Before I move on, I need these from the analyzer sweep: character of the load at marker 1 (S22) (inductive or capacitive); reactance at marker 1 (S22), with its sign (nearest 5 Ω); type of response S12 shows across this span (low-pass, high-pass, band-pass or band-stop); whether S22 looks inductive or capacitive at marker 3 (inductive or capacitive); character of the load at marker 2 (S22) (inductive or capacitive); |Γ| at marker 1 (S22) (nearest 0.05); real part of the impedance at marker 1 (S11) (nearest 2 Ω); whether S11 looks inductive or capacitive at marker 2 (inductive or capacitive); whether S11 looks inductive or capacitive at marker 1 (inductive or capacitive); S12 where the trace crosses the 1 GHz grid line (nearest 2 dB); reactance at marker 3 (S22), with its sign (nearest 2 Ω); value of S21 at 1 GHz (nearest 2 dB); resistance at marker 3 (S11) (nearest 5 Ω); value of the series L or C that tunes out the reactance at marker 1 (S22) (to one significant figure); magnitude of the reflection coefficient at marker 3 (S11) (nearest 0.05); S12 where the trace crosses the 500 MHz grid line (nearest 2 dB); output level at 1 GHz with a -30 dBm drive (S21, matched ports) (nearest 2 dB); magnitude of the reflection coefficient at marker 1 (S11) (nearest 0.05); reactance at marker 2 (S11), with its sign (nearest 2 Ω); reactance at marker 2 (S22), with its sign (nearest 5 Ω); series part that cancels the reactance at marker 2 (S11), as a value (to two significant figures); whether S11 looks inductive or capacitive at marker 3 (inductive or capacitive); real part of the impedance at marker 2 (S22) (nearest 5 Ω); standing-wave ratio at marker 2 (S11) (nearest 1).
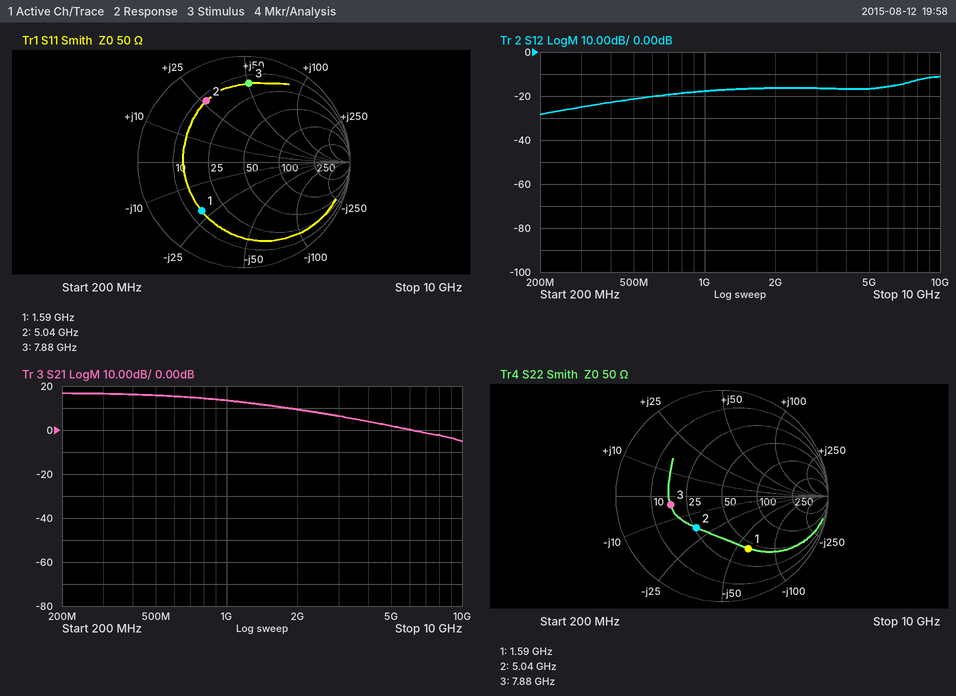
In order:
capacitive
-60 Ω
high-pass
capacitive
capacitive
0.55
14 Ω
inductive
capacitive
-18 dB
-4 Ω
14 dB
15 Ω
6 nH
0.75
-22 dB
-16 dBm
0.60
+26 Ω
-20 Ω
1.2 pF
inductive
25 Ω
5
